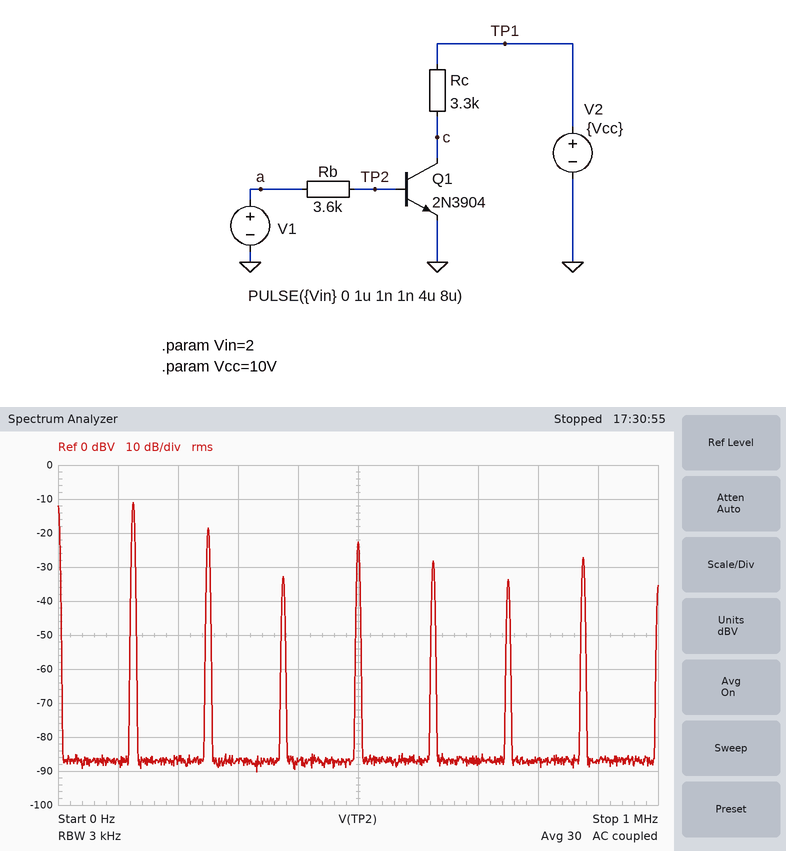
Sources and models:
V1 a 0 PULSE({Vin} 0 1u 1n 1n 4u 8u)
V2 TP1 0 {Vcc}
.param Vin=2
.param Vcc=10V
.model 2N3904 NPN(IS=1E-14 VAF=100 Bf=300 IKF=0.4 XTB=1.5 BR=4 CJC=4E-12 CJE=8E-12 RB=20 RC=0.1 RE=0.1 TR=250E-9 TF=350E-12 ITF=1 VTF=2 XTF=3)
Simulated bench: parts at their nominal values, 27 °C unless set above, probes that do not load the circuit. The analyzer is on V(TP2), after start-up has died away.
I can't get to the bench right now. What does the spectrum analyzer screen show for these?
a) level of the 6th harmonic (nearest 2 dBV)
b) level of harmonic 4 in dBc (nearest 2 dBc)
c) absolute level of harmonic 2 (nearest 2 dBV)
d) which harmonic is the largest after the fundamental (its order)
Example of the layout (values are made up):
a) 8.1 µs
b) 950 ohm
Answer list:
a) -34 dBV
b) -12 dBc
c) -18 dBV
d) 2
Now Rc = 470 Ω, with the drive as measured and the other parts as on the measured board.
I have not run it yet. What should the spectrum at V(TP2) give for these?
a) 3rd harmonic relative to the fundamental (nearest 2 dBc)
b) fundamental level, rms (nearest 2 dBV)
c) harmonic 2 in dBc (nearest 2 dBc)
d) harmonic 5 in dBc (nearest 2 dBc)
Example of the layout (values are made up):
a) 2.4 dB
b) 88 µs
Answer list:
a) -14 dBc
b) -10 dBV
c) -10 dBc
d) -38 dBc
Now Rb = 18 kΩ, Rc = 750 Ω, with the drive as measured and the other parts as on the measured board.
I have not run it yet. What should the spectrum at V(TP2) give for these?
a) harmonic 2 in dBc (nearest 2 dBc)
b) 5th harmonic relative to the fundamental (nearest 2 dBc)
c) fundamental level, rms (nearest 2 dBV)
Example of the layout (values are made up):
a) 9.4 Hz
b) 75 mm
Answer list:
a) -10 dBc
b) -30 dBc
c) -10 dBV
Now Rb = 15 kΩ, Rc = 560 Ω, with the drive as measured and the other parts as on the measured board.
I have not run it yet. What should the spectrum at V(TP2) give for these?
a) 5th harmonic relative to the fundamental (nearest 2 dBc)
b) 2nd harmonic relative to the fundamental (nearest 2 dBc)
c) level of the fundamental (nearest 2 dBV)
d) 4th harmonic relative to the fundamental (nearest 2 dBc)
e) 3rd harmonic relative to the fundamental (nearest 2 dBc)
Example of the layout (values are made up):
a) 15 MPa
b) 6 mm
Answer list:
a) -26 dBc
b) -12 dBc
c) -10 dBV
d) -14 dBc
e) -12 dBc
